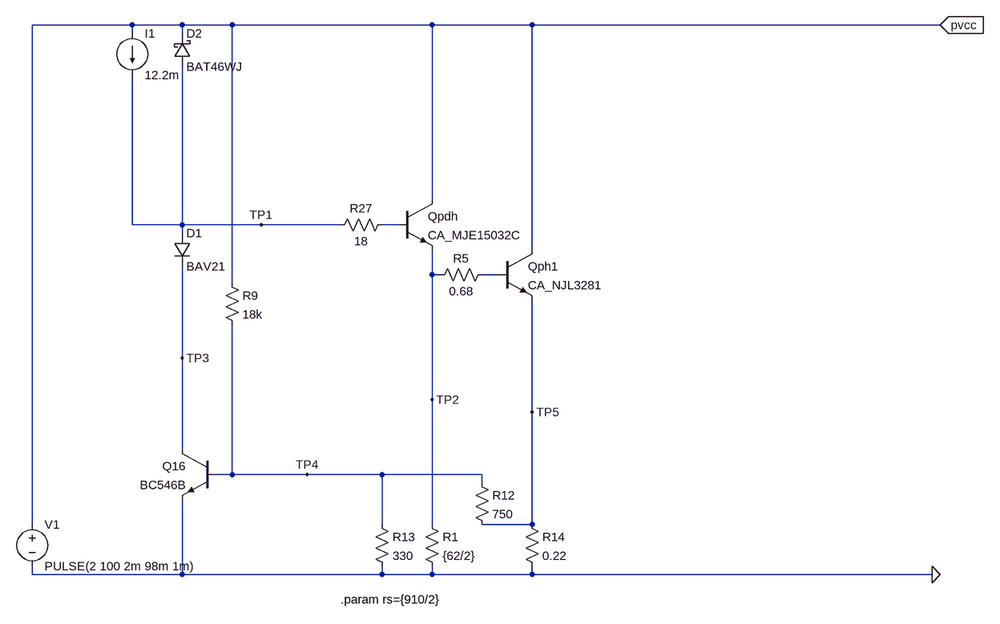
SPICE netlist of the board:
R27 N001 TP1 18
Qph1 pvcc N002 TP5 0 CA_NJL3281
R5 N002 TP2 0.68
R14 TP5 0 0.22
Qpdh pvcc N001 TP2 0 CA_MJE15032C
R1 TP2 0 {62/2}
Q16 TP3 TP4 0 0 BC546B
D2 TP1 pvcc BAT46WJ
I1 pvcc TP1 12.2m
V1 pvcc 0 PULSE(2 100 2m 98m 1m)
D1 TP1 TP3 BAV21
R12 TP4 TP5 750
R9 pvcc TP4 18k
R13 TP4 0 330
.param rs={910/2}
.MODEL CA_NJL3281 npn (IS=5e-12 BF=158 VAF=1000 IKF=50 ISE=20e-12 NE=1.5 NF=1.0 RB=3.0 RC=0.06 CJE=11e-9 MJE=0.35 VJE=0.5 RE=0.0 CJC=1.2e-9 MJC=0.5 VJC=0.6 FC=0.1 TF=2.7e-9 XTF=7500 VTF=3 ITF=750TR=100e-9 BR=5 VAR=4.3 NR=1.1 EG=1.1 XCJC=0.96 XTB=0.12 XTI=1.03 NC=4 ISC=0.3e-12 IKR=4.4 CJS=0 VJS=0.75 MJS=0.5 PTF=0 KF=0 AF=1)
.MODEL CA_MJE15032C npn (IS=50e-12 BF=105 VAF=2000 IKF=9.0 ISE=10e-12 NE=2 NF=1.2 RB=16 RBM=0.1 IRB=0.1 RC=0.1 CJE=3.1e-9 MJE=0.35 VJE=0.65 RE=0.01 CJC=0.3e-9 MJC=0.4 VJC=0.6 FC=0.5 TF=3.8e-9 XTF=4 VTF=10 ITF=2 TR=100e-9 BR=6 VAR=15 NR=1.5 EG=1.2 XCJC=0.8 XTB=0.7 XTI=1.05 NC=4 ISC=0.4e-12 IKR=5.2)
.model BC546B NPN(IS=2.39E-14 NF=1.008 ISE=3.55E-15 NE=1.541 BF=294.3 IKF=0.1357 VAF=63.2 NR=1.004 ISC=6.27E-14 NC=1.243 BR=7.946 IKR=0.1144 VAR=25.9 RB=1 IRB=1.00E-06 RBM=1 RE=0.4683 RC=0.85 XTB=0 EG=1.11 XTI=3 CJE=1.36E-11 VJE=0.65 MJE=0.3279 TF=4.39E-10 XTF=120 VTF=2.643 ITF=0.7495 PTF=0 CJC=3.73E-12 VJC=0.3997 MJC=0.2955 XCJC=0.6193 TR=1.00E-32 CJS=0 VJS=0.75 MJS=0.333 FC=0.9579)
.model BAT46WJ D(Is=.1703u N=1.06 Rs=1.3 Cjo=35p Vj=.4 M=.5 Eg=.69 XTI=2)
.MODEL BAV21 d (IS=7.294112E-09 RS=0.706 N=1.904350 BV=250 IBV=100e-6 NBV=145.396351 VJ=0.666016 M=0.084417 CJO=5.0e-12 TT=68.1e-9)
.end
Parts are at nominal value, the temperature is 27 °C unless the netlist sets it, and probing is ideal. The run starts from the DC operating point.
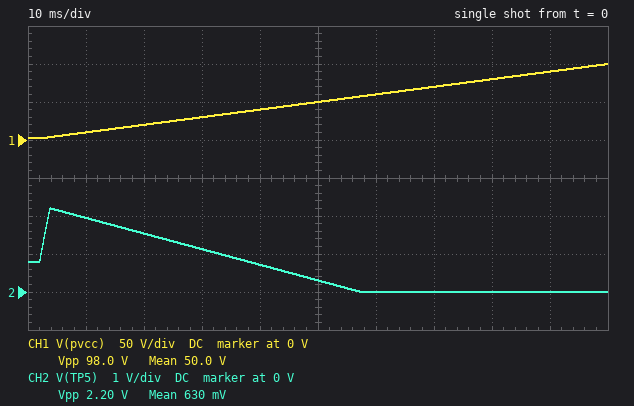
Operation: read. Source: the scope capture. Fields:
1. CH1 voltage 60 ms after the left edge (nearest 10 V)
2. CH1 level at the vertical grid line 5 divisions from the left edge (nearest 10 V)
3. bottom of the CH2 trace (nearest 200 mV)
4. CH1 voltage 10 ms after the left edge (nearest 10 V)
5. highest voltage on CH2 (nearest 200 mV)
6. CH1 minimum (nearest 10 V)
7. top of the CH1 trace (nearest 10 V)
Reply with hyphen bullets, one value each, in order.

- 60 V
- 50 V
- 0 V
- 10 V
- 2.2 V
- 0 V
- 100 V
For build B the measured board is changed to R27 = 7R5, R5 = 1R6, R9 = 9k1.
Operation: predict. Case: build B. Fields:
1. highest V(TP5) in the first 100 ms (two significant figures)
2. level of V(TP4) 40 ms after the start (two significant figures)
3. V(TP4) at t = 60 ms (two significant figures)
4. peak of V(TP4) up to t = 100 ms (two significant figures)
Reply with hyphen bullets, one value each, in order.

- 2.1 V
- 730 mV
- 750 mV
- 770 mV
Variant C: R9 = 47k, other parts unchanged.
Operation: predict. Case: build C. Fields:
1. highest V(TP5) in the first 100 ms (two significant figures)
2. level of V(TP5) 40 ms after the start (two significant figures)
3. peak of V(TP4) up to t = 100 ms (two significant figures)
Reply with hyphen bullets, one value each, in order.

- 2.3 V
- 1.7 V
- 710 mV
